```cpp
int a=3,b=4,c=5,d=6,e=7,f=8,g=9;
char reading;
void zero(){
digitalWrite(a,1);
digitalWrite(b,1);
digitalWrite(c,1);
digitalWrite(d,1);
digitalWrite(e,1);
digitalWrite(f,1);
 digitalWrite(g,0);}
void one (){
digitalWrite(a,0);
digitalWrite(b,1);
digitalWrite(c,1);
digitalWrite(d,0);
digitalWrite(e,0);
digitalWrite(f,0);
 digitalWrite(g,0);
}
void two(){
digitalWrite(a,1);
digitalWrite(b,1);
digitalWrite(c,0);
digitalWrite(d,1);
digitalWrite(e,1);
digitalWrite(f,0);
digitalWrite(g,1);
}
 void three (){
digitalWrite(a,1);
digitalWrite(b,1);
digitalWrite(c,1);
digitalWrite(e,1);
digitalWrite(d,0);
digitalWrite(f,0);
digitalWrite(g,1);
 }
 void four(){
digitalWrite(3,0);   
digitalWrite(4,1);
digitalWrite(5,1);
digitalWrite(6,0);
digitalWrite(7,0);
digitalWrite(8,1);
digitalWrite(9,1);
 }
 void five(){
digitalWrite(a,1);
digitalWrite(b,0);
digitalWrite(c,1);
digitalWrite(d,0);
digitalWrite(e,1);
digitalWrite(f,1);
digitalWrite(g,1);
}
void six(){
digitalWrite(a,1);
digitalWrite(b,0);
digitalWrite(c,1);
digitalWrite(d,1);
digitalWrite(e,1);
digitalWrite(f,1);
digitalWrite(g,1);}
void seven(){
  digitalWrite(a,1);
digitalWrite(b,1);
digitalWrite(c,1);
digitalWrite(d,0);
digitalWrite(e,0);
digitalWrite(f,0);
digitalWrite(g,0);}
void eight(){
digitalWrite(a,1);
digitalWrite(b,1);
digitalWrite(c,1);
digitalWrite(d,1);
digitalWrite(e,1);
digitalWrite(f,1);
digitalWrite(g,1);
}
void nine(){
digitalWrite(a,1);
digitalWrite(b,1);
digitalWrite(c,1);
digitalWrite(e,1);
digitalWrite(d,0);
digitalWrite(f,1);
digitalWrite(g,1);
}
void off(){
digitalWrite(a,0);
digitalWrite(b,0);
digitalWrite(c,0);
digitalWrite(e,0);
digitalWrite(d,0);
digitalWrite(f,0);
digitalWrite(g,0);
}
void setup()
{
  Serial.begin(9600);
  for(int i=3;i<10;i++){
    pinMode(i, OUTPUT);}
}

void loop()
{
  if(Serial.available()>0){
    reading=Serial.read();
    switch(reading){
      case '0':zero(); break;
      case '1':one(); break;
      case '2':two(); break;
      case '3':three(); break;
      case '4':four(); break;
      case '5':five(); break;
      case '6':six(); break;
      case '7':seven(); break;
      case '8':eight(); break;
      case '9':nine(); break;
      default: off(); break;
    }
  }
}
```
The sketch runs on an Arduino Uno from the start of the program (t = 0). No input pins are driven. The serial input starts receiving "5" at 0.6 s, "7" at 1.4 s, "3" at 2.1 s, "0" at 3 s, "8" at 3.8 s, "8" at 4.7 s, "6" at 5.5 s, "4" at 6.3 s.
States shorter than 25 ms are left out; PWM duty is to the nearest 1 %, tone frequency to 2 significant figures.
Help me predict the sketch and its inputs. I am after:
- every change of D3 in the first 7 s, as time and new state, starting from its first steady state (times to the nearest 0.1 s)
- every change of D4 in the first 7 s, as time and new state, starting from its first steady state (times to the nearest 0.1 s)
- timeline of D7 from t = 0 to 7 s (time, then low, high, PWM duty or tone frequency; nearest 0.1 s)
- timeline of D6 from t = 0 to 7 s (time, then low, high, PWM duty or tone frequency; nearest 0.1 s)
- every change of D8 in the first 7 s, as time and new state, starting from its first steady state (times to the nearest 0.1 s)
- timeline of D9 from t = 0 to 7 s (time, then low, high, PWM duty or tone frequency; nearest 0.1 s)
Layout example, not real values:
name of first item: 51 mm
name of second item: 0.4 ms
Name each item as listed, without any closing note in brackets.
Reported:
every change of D3 in the first 7 s, as time and new state, starting from its first steady state: 0 s low; 0.6 s high; 6.3 s low
every change of D4 in the first 7 s, as time and new state, starting from its first steady state: 0 s low; 1.4 s high; 5.5 s low; 6.3 s high
timeline of D7 from t = 0 to 7 s: 0 s low; 0.6 s high; 1.4 s low; 2.1 s high; 6.3 s low
timeline of D6 from t = 0 to 7 s: 0 s low; 3 s high; 6.3 s low
every change of D8 in the first 7 s, as time and new state, starting from its first steady state: 0 s low; 0.6 s high; 1.4 s low; 3 s high
timeline of D9 from t = 0 to 7 s: 0 s low; 0.6 s high; 1.4 s low; 2.1 s high; 3 s low; 3.8 s high
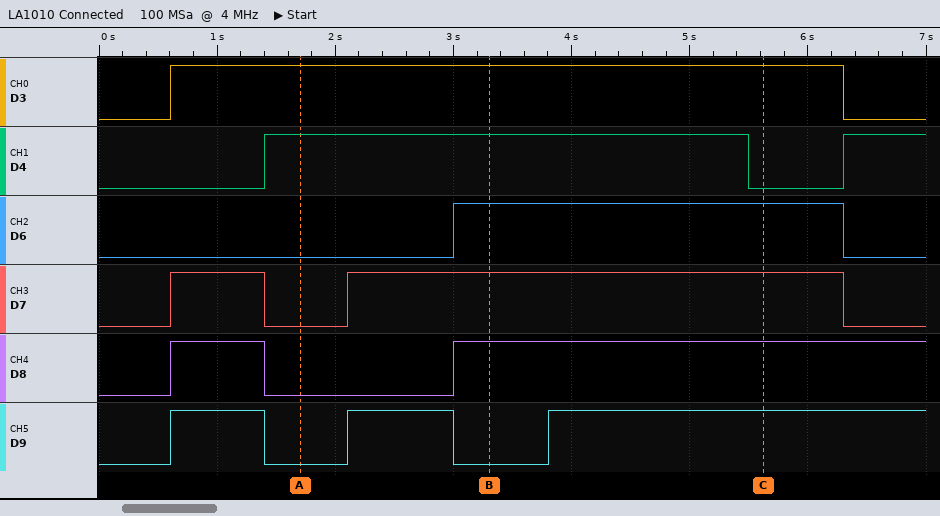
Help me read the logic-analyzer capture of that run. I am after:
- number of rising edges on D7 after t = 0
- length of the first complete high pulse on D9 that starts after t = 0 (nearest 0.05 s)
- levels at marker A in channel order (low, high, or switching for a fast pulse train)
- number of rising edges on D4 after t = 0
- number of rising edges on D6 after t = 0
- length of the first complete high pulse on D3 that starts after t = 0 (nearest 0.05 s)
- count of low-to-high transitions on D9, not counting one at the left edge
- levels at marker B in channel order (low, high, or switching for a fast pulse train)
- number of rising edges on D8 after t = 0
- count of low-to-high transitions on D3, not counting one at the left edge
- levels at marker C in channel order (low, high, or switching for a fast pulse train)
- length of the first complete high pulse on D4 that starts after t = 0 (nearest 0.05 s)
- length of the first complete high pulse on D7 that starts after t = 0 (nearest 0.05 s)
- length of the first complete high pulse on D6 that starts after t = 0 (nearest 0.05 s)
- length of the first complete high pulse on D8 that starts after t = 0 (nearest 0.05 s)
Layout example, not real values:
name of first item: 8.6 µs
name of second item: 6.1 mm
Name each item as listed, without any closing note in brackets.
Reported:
number of rising edges on D7 after t = 0: 2
length of the first complete high pulse on D9 that starts after t = 0: 0.80 s
levels at marker A in channel order: D3 high, D4 high, D6 low, D7 low, D8 low, D9 low
number of rising edges on D4 after t = 0: 2
number of rising edges on D6 after t = 0: 1
length of the first complete high pulse on D3 that starts after t = 0: 5.70 s
count of low-to-high transitions on D9, not counting one at the left edge: 3
levels at marker B in channel order: D3 high, D4 high, D6 high, D7 high, D8 high, D9 low
number of rising edges on D8 after t = 0: 2
count of low-to-high transitions on D3, not counting one at the left edge: 1
levels at marker C in channel order: D3 high, D4 low, D6 high, D7 high, D8 high, D9 high
length of the first complete high pulse on D4 that starts after t = 0: 4.10 s
length of the first complete high pulse on D7 that starts after t = 0: 0.80 s
length of the first complete high pulse on D6 that starts after t = 0: 3.30 s
length of the first complete high pulse on D8 that starts after t = 0: 0.80 s
